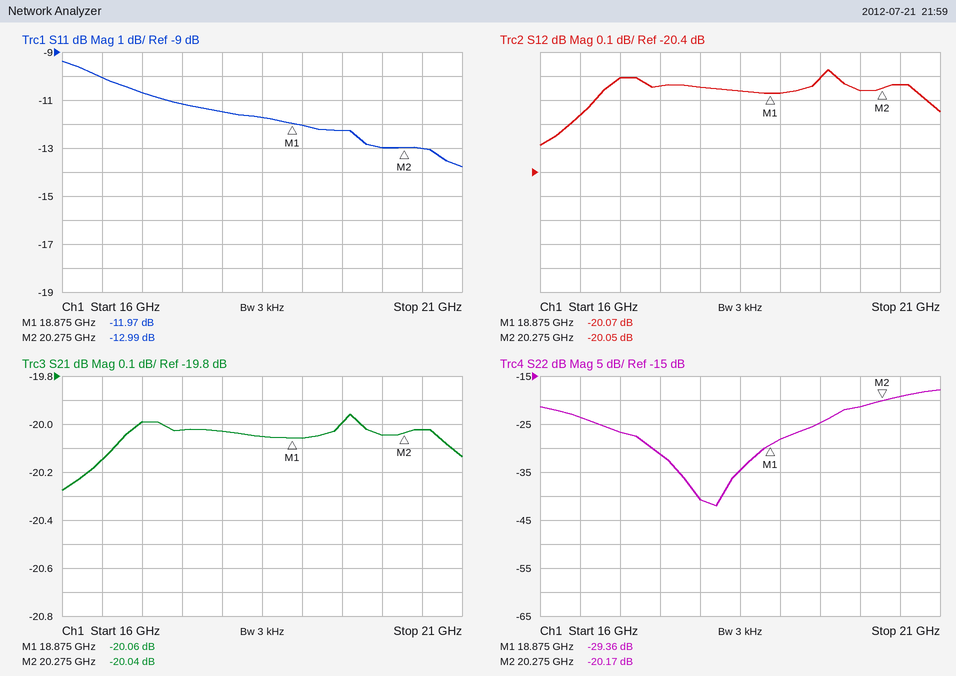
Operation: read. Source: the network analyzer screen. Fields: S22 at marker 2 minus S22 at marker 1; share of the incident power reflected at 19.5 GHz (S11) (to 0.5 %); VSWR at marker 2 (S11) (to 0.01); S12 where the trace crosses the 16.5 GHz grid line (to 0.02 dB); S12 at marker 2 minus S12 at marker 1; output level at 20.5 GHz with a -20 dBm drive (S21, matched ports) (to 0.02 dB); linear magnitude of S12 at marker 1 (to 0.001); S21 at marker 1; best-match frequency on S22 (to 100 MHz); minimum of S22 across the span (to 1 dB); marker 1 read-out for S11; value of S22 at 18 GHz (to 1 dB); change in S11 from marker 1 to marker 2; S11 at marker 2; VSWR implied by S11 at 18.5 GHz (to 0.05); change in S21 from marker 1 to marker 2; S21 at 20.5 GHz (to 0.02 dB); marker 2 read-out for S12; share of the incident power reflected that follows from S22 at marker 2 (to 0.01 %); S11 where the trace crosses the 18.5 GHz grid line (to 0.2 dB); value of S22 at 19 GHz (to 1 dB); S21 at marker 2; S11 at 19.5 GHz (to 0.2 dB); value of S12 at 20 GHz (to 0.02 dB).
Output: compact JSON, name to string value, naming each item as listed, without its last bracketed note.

{"S22 at marker 2 minus S22 at marker 1": "9.19 dB", "share of the incident power reflected at 19.5 GHz (S11)": "6.0 %", "VSWR at marker 2 (S11)": "1.58", "S12 where the trace crosses the 16.5 GHz grid line": "-20.16 dB", "S12 at marker 2 minus S12 at marker 1": "0.02 dB", "output level at 20.5 GHz with a -20 dBm drive (S21, matched ports)": "-40.02 dBm", "linear magnitude of S12 at marker 1": "0.099", "S21 at marker 1": "-20.06 dB", "best-match frequency on S22": "18.2 GHz", "minimum of S22 across the span": "-42 dB", "marker 1 read-out for S11": "-11.97 dB", "value of S22 at 18 GHz": "-41 dB", "change in S11 from marker 1 to marker 2": "-1.02 dB", "S11 at marker 2": "-12.99 dB", "VSWR implied by S11 at 18.5 GHz": "1.70", "change in S21 from marker 1 to marker 2": "0.02 dB", "S21 at 20.5 GHz": "-20.02 dB", "marker 2 read-out for S12": "-20.05 dB", "share of the incident power reflected that follows from S22 at marker 2": "0.96 %", "S11 where the trace crosses the 18.5 GHz grid line": "-11.8 dB", "value of S22 at 19 GHz": "-28 dB", "S21 at marker 2": "-20.04 dB", "S11 at 19.5 GHz": "-12.2 dB", "value of S12 at 20 GHz": "-20.06 dB"}
